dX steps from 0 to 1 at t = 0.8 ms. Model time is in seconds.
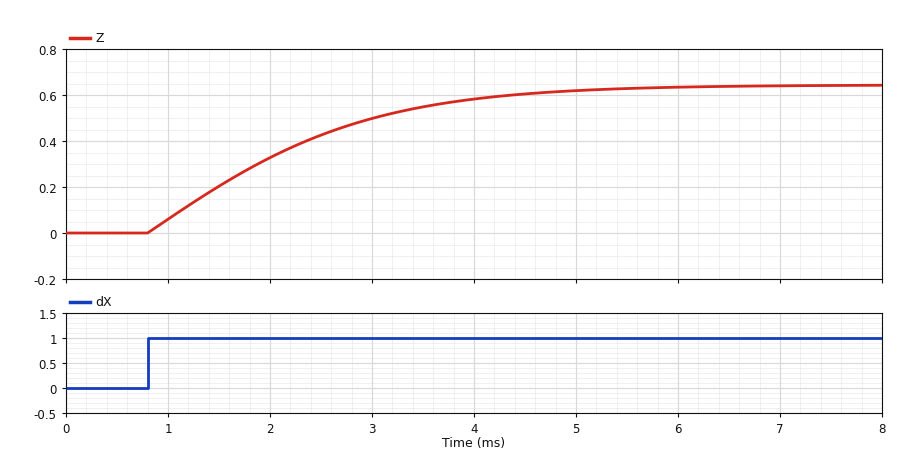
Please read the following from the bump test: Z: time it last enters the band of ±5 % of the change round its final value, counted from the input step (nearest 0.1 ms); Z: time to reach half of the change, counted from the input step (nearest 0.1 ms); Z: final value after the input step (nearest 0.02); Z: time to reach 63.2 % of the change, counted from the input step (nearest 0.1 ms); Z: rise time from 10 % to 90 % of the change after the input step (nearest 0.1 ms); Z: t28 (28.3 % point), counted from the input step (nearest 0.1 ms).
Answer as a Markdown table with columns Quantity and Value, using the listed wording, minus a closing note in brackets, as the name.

| Quantity | Value |
|---|---|
| Z: time it last enters the band of ±5 % of the change round its final value, counted from the input step | 3.9 ms |
| Z: time to reach half of the change, counted from the input step | 1.2 ms |
| Z: final value after the input step | 0.64 |
| Z: time to reach 63.2 % of the change, counted from the input step | 1.6 ms |
| Z: rise time from 10 % to 90 % of the change after the input step | 2.9 ms |
| Z: t28 (28.3 % point), counted from the input step | 0.6 ms |
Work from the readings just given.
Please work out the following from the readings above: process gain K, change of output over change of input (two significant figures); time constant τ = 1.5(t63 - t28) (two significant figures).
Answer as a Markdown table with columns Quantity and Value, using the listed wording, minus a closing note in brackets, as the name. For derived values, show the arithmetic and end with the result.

| Quantity | Value |
|---|---|
| process gain K, change of output over change of input | (0.64 - 0) / 1 = 0.64 |
| time constant τ = 1.5(t63 - t28) | 1.5 × (1.6 - 0.6) = 1.5 ms |
